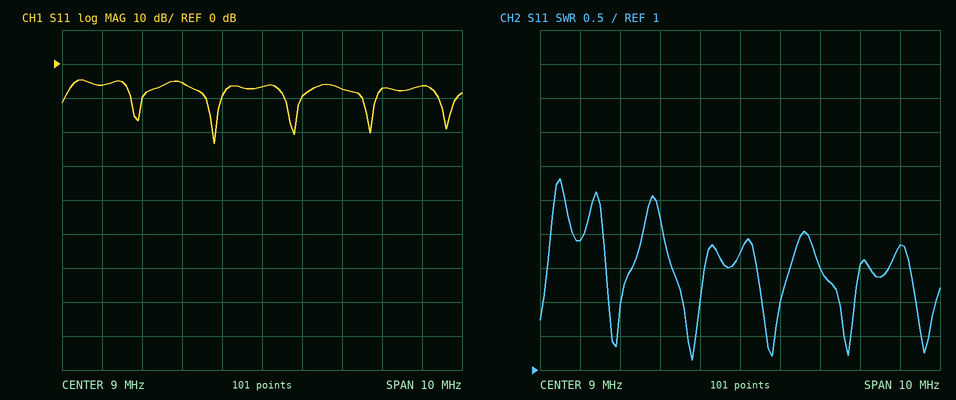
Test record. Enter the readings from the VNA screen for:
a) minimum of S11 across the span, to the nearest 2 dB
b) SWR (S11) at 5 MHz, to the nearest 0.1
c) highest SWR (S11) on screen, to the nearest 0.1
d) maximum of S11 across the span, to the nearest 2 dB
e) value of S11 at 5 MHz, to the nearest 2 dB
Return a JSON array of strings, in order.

["-24 dB", "2.9", "3.8", "-4 dB", "-6 dB"]
